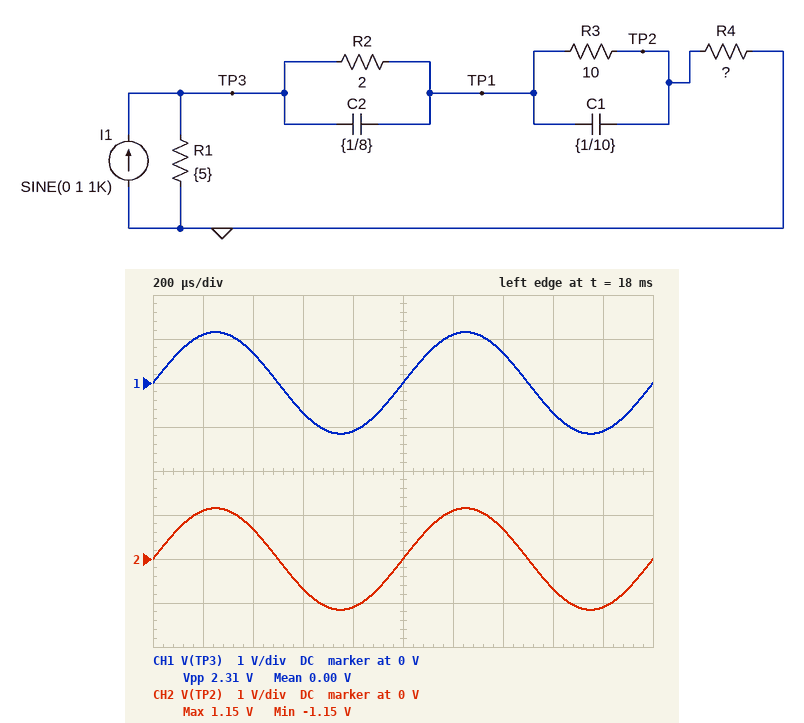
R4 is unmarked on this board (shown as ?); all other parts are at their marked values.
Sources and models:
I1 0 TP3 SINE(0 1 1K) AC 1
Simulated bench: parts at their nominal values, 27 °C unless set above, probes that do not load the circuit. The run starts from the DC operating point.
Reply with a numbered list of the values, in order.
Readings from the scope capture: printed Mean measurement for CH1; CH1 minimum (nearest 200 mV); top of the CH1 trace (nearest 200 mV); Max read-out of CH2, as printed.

1. 0.00 V
2. -1.2 V
3. 1.2 V
4. 1.15 V
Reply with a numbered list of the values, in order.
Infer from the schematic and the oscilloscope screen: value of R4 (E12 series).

1. 1.5 Ω
